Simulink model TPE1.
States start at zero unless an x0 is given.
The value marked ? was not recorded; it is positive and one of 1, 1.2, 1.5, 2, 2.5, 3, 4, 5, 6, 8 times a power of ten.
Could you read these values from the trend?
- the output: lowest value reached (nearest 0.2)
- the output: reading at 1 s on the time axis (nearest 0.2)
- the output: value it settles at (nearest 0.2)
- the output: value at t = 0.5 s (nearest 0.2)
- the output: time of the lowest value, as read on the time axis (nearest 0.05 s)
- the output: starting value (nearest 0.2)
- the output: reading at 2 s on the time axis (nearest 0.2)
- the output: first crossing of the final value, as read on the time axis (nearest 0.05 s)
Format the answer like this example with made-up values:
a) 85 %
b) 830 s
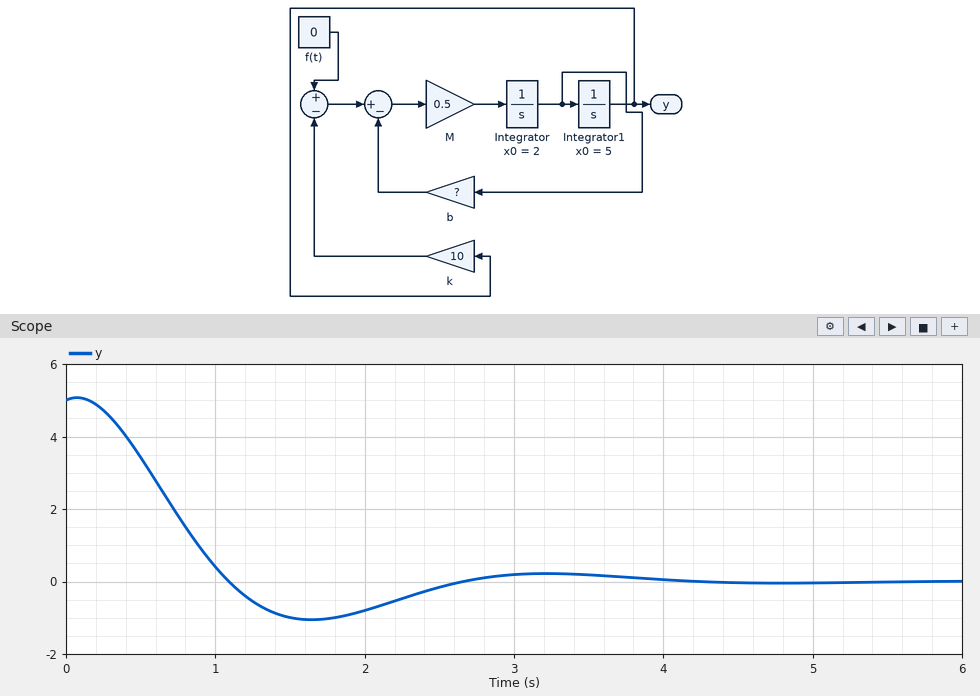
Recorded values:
a) -1.0
b) 0.4
c) 0.0
d) 3.4
e) 1.65 s
f) 5.0
g) -0.8
h) 1.10 s
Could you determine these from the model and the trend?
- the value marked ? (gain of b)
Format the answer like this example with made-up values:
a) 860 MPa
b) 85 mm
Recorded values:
a) 4
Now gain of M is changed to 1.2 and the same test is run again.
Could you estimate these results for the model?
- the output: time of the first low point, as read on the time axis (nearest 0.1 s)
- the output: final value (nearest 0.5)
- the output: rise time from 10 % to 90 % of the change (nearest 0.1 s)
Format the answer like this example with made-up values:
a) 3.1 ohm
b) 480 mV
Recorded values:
a) 1.3 s
b) 0.0
c) 0.6 s
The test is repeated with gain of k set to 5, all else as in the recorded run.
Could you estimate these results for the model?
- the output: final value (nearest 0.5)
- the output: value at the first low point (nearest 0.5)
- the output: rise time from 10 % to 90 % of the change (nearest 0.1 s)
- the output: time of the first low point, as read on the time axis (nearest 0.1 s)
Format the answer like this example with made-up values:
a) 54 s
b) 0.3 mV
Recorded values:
a) 0.0
b) -0.5
c) 1.2 s
d) 2.7 s
